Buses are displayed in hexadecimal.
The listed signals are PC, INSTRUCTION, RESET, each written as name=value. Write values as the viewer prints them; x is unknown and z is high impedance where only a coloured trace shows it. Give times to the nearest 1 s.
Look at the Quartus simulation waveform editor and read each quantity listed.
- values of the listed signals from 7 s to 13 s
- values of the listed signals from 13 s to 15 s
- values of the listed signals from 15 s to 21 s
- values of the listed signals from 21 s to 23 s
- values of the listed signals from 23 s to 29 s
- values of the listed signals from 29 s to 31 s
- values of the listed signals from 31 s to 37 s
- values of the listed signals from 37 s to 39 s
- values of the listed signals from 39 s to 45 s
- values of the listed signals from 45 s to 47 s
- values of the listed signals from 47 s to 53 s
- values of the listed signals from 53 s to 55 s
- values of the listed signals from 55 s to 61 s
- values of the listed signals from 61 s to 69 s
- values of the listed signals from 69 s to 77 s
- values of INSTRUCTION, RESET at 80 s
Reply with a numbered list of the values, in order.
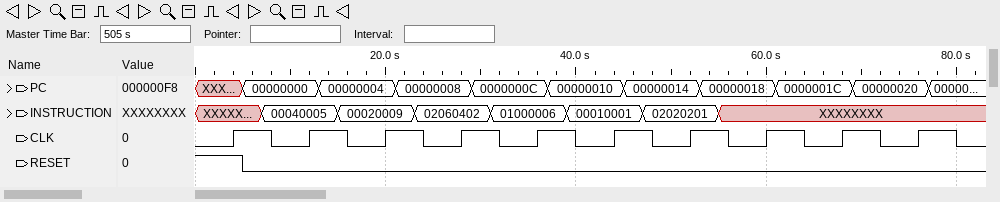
1. PC=00000000, INSTRUCTION=00040005, RESET=0
2. PC=00000004, INSTRUCTION=00040005, RESET=0
3. PC=00000004, INSTRUCTION=00020009, RESET=0
4. PC=00000008, INSTRUCTION=00020009, RESET=0
5. PC=00000008, INSTRUCTION=02060402, RESET=0
6. PC=0000000C, INSTRUCTION=02060402, RESET=0
7. PC=0000000C, INSTRUCTION=01000006, RESET=0
8. PC=00000010, INSTRUCTION=01000006, RESET=0
9. PC=00000010, INSTRUCTION=00010001, RESET=0
10. PC=00000014, INSTRUCTION=00010001, RESET=0
11. PC=00000014, INSTRUCTION=02020201, RESET=0
12. PC=00000018, INSTRUCTION=02020201, RESET=0
13. PC=00000018, INSTRUCTION=XXXXXXXX, RESET=0
14. PC=0000001C, INSTRUCTION=XXXXXXXX, RESET=0
15. PC=00000020, INSTRUCTION=XXXXXXXX, RESET=0
16. INSTRUCTION=XXXXXXXX, RESET=0
